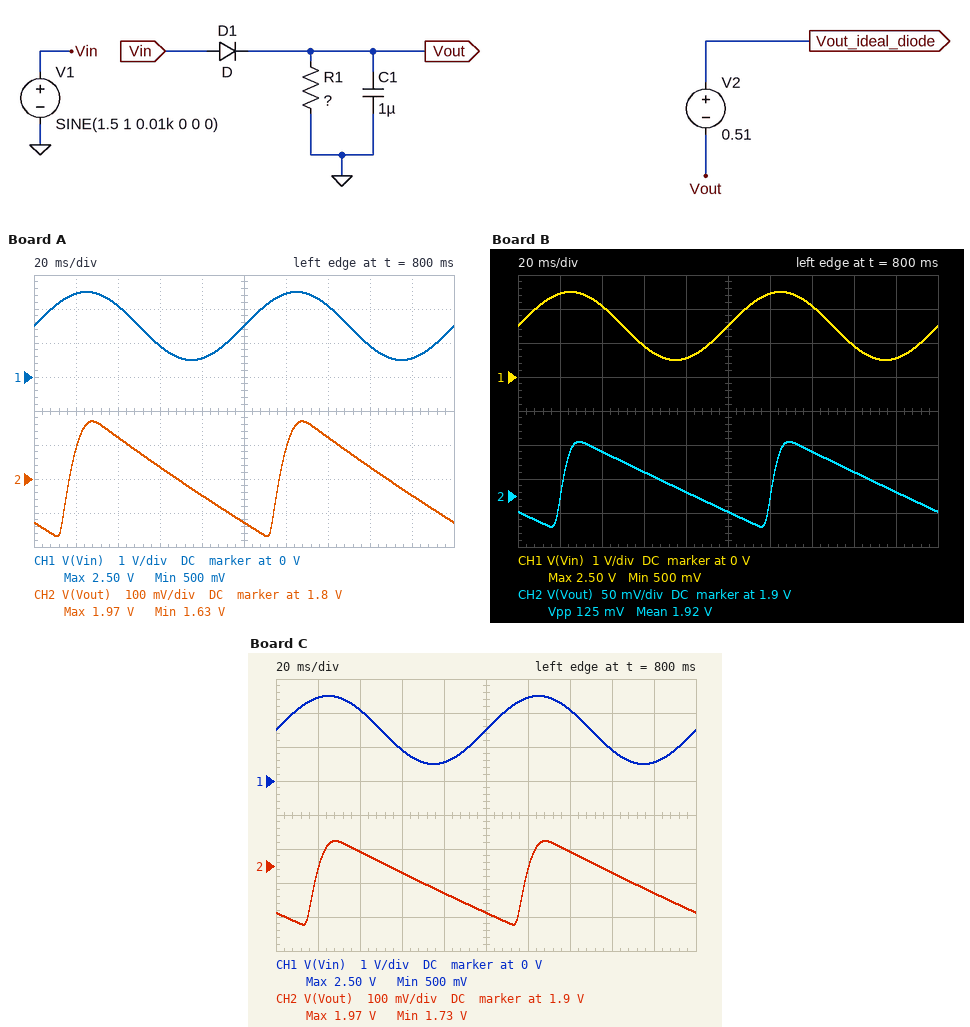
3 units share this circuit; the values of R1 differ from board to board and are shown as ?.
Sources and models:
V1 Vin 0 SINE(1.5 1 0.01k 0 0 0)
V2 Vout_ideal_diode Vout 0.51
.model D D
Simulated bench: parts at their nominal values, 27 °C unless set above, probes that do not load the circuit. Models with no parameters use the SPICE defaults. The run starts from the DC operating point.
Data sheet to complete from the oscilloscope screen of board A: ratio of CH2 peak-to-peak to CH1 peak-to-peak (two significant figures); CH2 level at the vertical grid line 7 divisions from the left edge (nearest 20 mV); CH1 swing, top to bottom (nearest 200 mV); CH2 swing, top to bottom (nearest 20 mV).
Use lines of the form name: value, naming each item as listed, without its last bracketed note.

ratio of CH2 peak-to-peak to CH1 peak-to-peak: 0.17
CH2 level at the vertical grid line 7 divisions from the left edge: 1.92 V
CH1 swing, top to bottom: 2.0 V
CH2 swing, top to bottom: 340 mV
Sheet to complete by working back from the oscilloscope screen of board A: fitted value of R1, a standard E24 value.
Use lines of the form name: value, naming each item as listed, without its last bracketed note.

fitted value of R1, a standard E24 value: 430 kΩ
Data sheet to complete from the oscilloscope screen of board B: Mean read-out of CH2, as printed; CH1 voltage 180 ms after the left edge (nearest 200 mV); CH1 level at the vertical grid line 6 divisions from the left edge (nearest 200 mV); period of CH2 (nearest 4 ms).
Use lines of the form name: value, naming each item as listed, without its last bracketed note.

Mean read-out of CH2, as printed: 1.92 V
CH1 voltage 180 ms after the left edge: 600 mV
CH1 level at the vertical grid line 6 divisions from the left edge: 2.4 V
period of CH2: 100 ms
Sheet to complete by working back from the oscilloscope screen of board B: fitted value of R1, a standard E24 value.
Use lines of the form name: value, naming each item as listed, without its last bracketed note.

fitted value of R1, a standard E24 value: 1.3 MΩ
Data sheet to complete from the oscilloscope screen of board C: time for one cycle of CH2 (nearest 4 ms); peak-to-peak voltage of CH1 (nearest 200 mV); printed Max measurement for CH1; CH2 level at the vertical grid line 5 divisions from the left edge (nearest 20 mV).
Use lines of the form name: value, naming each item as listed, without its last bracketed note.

time for one cycle of CH2: 100 ms
peak-to-peak voltage of CH1: 2.0 V
printed Max measurement for CH1: 2.50 V
CH2 level at the vertical grid line 5 divisions from the left edge: 1.76 V
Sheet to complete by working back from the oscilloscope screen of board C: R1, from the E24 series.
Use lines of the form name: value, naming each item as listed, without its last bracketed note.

R1, from the E24 series: 620 kΩ
